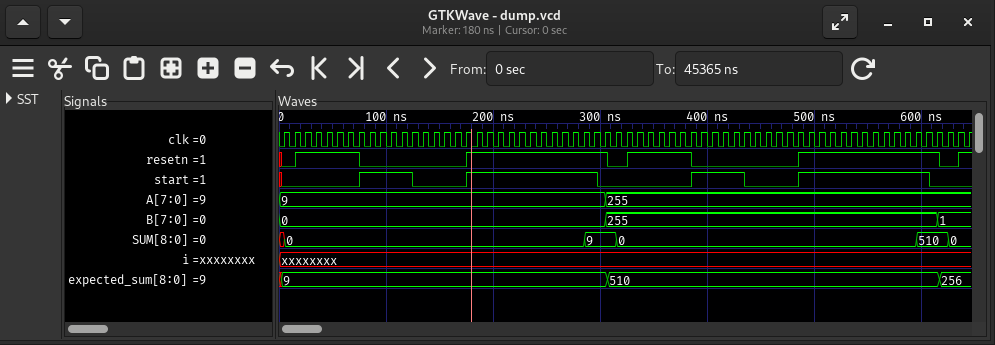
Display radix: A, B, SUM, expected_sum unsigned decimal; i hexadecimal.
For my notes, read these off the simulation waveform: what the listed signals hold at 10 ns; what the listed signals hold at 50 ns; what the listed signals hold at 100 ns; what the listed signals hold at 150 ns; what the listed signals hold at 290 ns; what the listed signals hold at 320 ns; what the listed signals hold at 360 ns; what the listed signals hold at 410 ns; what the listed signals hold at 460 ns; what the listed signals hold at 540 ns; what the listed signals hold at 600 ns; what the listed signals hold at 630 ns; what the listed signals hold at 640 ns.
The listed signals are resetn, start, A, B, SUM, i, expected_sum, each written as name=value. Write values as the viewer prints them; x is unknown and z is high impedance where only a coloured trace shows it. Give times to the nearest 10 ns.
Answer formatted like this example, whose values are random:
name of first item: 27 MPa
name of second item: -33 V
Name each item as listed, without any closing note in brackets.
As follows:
what the listed signals hold at 10 ns: resetn=0, start=0, A=9, B=0, SUM=0, i=xxxxxxxx, expected_sum=9
what the listed signals hold at 50 ns: resetn=1, start=0, A=9, B=0, SUM=0, i=xxxxxxxx, expected_sum=9
what the listed signals hold at 100 ns: resetn=0, start=1, A=9, B=0, SUM=0, i=xxxxxxxx, expected_sum=9
what the listed signals hold at 150 ns: resetn=0, start=0, A=9, B=0, SUM=0, i=xxxxxxxx, expected_sum=9
what the listed signals hold at 290 ns: resetn=1, start=1, A=9, B=0, SUM=9, i=xxxxxxxx, expected_sum=9
what the listed signals hold at 320 ns: resetn=0, start=0, A=255, B=255, SUM=0, i=xxxxxxxx, expected_sum=510
what the listed signals hold at 360 ns: resetn=1, start=0, A=255, B=255, SUM=0, i=xxxxxxxx, expected_sum=510
what the listed signals hold at 410 ns: resetn=0, start=1, A=255, B=255, SUM=0, i=xxxxxxxx, expected_sum=510
what the listed signals hold at 460 ns: resetn=0, start=0, A=255, B=255, SUM=0, i=xxxxxxxx, expected_sum=510
what the listed signals hold at 540 ns: resetn=1, start=1, A=255, B=255, SUM=0, i=xxxxxxxx, expected_sum=510
what the listed signals hold at 600 ns: resetn=1, start=1, A=255, B=255, SUM=510, i=xxxxxxxx, expected_sum=510
what the listed signals hold at 630 ns: resetn=0, start=0, A=255, B=1, SUM=0, i=xxxxxxxx, expected_sum=256
what the listed signals hold at 640 ns: resetn=1, start=0, A=255, B=1, SUM=0, i=xxxxxxxx, expected_sum=256
